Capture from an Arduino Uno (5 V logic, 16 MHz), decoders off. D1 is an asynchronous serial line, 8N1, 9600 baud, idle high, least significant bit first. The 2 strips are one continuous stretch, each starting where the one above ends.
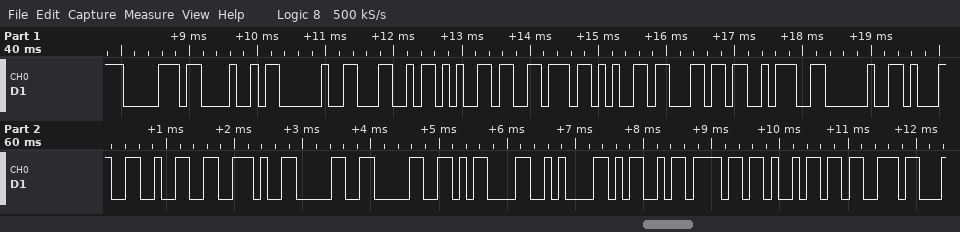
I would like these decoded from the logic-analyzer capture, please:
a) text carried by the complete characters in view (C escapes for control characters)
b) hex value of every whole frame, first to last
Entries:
"pH Level: 12.00\r\nMois"
70 48 20 4C 65 76 65 6C 3A 20 31 32 2E 30 30 0D 0A 4D 6F 69 73
